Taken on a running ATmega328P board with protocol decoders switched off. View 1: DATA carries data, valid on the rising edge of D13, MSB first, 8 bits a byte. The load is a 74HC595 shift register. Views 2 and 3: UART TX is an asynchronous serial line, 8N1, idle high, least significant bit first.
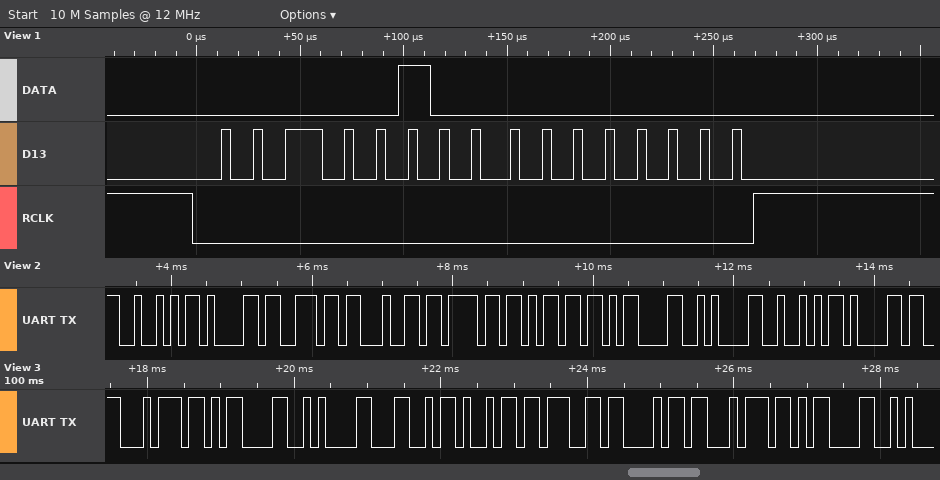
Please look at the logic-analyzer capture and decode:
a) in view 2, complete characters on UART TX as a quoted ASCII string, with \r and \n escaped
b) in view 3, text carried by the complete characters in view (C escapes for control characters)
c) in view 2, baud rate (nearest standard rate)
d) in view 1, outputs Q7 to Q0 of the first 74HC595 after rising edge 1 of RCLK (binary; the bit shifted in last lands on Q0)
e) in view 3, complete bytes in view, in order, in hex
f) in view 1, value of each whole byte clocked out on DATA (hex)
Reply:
"Random\r\nRa"
"t\r\nLight\r"
9600 baud
00000000
0x74 0x0D 0x0A 0x4C 0x69 0x67 0x68 0x74 0x0D
0x04 0x00
